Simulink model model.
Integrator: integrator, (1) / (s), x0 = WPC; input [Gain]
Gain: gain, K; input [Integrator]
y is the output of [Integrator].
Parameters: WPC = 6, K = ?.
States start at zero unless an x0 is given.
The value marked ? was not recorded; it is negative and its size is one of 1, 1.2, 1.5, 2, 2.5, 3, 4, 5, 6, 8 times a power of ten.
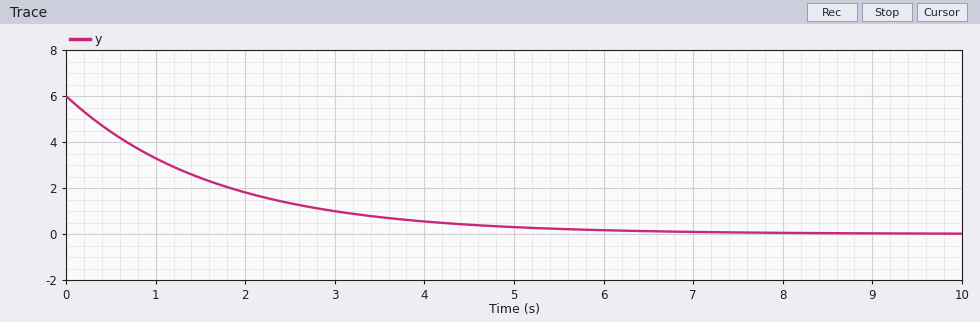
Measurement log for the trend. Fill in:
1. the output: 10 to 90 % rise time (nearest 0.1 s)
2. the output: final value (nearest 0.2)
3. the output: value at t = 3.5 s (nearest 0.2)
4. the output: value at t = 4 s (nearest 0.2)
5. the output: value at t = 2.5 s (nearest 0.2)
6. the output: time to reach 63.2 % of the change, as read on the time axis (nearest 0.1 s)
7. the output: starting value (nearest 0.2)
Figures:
3.7 s
0.0
0.8
0.6
1.4
1.7 s
6.0
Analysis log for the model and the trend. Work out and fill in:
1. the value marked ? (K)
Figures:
-0.6
